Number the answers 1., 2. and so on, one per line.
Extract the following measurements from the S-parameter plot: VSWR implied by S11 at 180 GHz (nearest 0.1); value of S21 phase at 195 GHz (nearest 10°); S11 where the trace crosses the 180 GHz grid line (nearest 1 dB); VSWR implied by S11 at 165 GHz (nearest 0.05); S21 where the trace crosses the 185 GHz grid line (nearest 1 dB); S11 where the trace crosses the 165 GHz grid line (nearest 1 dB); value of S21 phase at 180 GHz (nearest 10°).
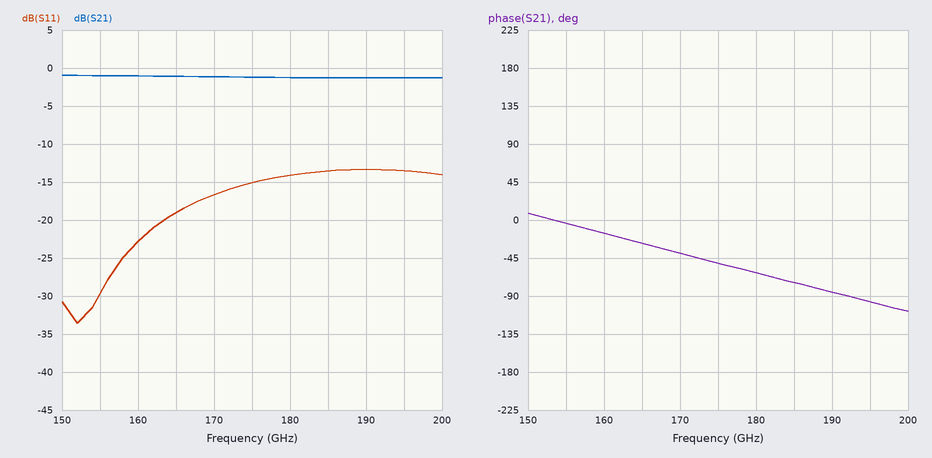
1. 1.5
2. -100°
3. -14 dB
4. 1.25
5. -1 dB
6. -19 dB
7. -60°
